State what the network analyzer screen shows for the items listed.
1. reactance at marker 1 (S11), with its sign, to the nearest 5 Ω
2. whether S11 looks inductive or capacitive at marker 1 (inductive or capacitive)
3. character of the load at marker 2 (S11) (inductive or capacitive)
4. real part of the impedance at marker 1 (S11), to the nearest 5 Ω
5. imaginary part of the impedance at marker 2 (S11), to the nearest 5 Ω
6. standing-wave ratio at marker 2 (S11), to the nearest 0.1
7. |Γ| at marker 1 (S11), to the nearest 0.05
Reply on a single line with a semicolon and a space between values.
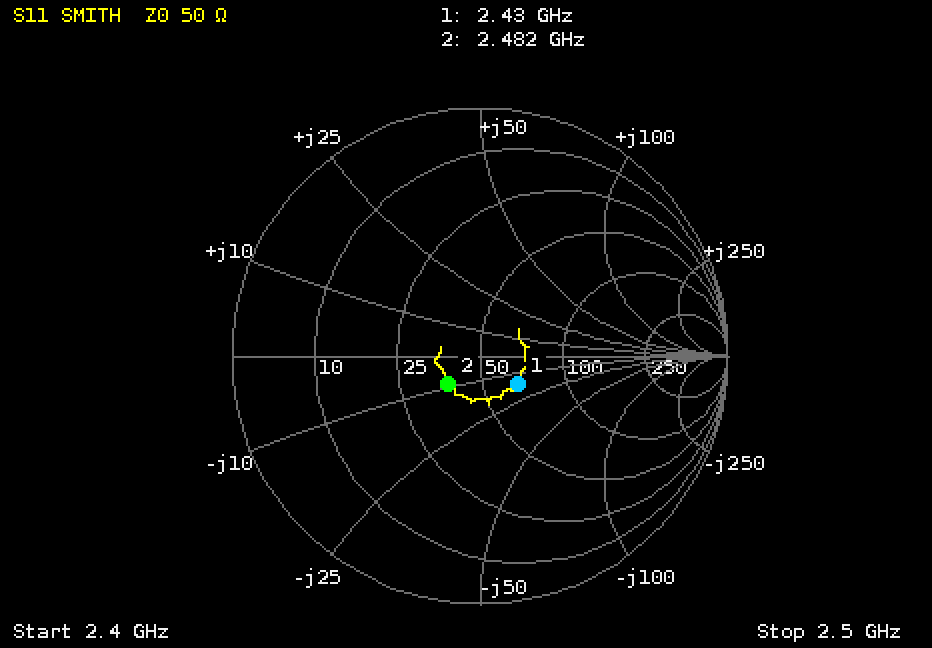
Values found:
-15 Ω; capacitive; capacitive; 65 Ω; -10 Ω; 1.4; 0.20
